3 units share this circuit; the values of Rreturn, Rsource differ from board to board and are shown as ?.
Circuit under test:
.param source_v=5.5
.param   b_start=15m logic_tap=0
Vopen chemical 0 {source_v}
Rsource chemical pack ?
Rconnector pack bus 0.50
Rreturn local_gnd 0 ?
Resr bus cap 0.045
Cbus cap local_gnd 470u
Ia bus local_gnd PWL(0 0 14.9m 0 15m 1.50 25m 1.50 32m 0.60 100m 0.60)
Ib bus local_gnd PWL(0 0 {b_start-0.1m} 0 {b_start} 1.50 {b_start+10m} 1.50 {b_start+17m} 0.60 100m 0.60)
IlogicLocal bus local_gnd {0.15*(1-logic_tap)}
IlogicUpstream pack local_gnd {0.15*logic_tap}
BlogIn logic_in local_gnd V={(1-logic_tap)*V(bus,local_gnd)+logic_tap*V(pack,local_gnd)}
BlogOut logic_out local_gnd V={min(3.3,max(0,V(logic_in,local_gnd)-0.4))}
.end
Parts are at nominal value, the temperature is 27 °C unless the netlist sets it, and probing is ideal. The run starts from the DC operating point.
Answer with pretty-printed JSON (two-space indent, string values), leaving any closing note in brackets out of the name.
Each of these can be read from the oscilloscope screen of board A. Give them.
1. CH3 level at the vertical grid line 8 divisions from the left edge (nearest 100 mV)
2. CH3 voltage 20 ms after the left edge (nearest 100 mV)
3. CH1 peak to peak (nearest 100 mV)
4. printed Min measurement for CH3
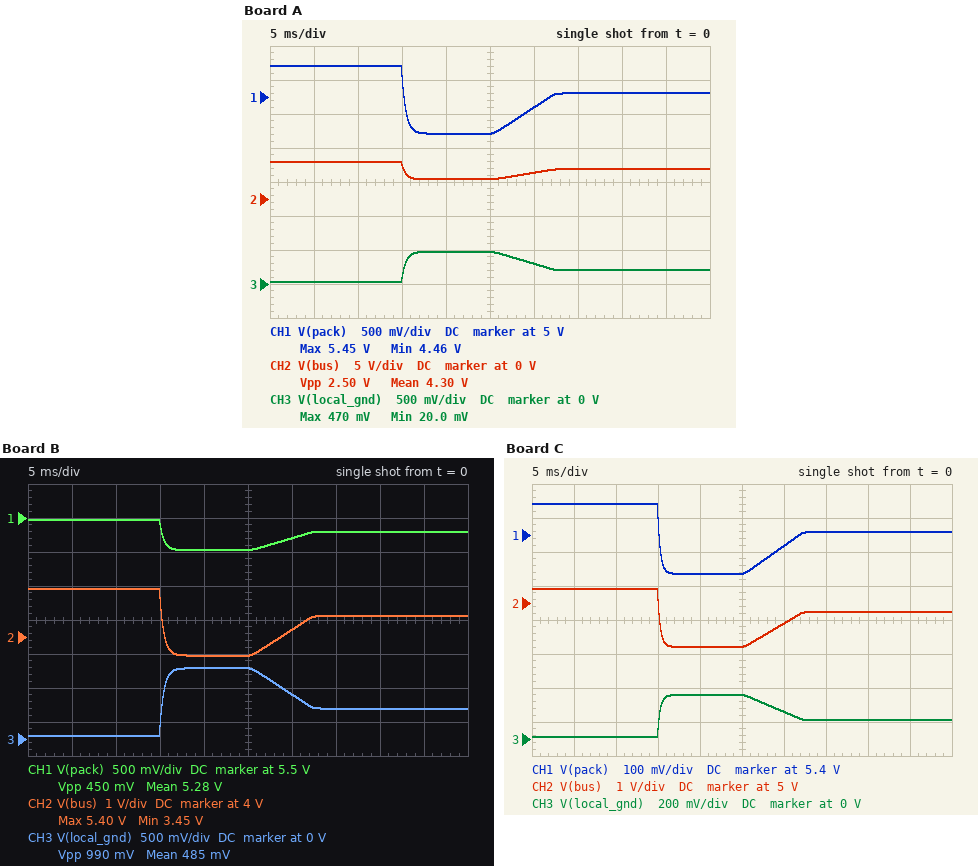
{
  "CH3 level at the vertical grid line 8 divisions from the left edge": "200 mV",
  "CH3 voltage 20 ms after the left edge": "500 mV",
  "CH1 peak to peak": "1.0 V",
  "printed Min measurement for CH3": "20.0 mV"
}
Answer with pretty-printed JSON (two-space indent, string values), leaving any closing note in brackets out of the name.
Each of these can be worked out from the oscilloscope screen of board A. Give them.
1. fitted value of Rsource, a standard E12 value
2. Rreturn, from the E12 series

{
  "fitted value of Rsource, a standard E12 value": "0.33 Ω",
  "Rreturn, from the E12 series": "0.15 Ω"
}
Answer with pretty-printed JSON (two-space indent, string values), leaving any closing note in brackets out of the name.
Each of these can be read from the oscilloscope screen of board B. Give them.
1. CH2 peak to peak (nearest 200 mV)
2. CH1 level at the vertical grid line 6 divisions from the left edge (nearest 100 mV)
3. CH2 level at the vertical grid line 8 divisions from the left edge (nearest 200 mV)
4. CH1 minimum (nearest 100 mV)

{
  "CH2 peak to peak": "2.0 V",
  "CH1 level at the vertical grid line 6 divisions from the left edge": "5.2 V",
  "CH2 level at the vertical grid line 8 divisions from the left edge": "4.6 V",
  "CH1 minimum": "5.0 V"
}
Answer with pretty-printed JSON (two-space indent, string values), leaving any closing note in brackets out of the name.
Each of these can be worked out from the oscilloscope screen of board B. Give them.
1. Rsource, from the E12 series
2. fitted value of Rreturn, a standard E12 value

{
  "Rsource, from the E12 series": "0.15 Ω",
  "fitted value of Rreturn, a standard E12 value": "0.33 Ω"
}
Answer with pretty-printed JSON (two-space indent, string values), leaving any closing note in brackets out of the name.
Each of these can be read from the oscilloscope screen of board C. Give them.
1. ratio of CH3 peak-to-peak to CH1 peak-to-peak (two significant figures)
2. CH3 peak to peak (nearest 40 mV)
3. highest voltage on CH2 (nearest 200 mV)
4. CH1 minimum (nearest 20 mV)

{
  "ratio of CH3 peak-to-peak to CH1 peak-to-peak": "1.2",
  "CH3 peak to peak": "240 mV",
  "highest voltage on CH2": "5.4 V",
  "CH1 minimum": "5.28 V"
}
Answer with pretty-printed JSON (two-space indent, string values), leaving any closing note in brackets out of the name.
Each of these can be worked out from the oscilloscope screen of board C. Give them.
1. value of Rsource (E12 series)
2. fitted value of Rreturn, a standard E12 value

{
  "value of Rsource": "0.068 Ω",
  "fitted value of Rreturn, a standard E12 value": "0.082 Ω"
}
